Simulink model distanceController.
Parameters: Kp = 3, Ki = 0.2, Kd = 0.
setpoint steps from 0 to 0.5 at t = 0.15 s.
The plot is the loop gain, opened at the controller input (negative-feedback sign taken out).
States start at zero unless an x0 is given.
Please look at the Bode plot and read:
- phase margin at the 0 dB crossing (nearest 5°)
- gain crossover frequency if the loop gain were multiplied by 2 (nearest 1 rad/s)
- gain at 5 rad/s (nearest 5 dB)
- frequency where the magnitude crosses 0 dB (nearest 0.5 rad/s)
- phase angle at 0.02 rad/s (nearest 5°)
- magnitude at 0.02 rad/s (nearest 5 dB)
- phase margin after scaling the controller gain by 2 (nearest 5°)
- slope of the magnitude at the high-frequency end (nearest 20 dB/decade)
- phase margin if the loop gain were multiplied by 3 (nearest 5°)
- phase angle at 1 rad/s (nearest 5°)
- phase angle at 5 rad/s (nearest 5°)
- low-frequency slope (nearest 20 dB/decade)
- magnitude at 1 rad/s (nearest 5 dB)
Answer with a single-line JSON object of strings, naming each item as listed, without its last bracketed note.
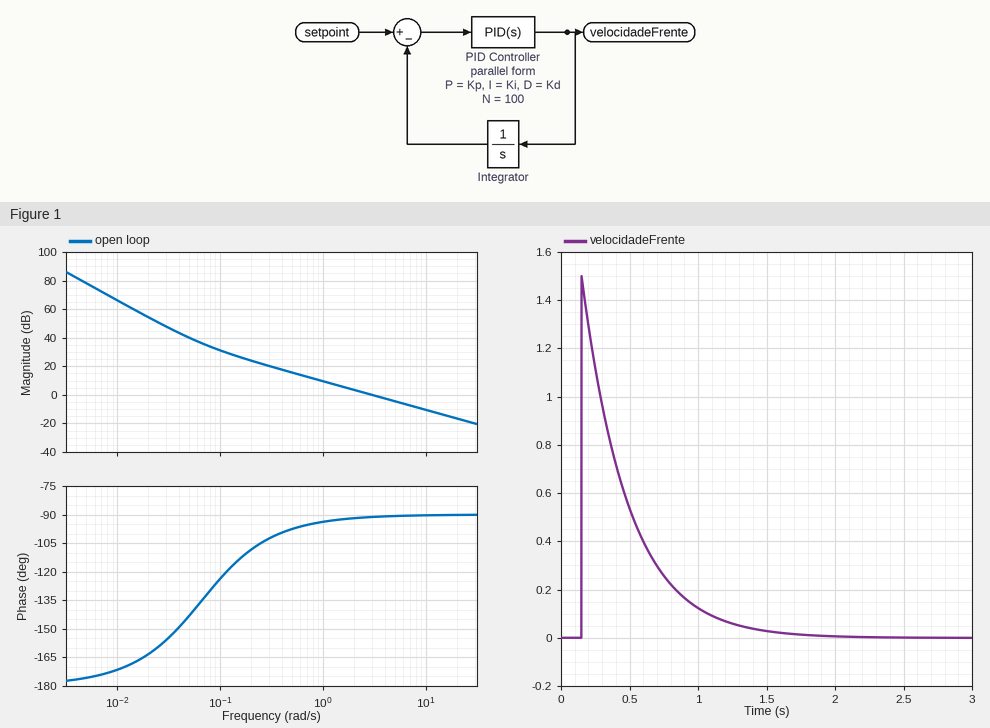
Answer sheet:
{"phase margin at the 0 dB crossing": "90°", "gain crossover frequency if the loop gain were multiplied by 2": "6 rad/s", "gain at 5 rad/s": "-5 dB", "frequency where the magnitude crosses 0 dB": "3.0 rad/s", "phase angle at 0.02 rad/s": "-165°", "magnitude at 0.02 rad/s": "55 dB", "phase margin after scaling the controller gain by 2": "90°", "slope of the magnitude at the high-frequency end": "-20 dB/decade", "phase margin if the loop gain were multiplied by 3": "90°", "phase angle at 1 rad/s": "-95°", "phase angle at 5 rad/s": "-90°", "low-frequency slope": "-40 dB/decade", "magnitude at 1 rad/s": "10 dB"}
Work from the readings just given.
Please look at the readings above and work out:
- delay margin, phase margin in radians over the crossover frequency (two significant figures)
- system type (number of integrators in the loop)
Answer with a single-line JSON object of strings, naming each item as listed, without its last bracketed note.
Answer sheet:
{"delay margin, phase margin in radians over the crossover frequency": "0.52 s", "system type": "2"}
